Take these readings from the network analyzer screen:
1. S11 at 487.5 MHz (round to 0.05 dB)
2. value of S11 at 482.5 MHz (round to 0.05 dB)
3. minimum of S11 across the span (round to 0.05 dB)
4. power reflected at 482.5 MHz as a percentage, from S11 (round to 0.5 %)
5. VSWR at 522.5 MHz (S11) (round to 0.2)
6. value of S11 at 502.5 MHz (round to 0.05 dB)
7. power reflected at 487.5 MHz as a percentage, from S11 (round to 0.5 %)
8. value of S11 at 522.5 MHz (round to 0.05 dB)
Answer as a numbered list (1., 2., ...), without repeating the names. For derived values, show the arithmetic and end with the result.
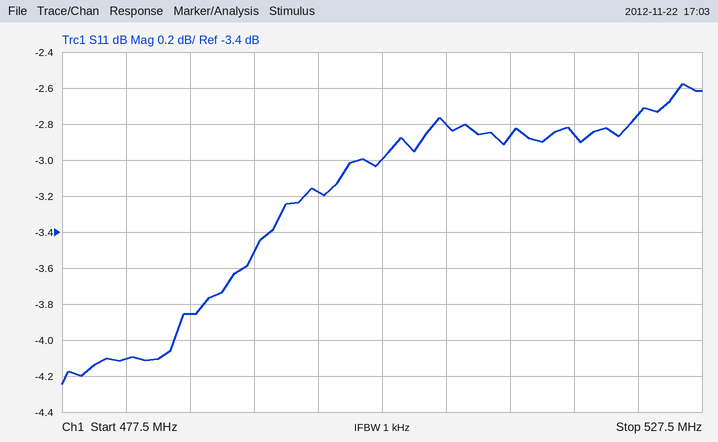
1. -3.85 dB
2. -4.10 dB
3. -4.25 dB
4. 10^(-4.1/10) ≈ 38.9 %, so 39.0 % to the nearest 0.5 %
5. |Γ| = 10^(-2.75/20) = 0.7286; VSWR = (1 + 0.7286)/(1 − 0.7286) ≈ 6.4
6. -3.00 dB
7. 10^(-3.85/10) ≈ 41.2 %, so 41.0 % to the nearest 0.5 %
8. -2.75 dB
